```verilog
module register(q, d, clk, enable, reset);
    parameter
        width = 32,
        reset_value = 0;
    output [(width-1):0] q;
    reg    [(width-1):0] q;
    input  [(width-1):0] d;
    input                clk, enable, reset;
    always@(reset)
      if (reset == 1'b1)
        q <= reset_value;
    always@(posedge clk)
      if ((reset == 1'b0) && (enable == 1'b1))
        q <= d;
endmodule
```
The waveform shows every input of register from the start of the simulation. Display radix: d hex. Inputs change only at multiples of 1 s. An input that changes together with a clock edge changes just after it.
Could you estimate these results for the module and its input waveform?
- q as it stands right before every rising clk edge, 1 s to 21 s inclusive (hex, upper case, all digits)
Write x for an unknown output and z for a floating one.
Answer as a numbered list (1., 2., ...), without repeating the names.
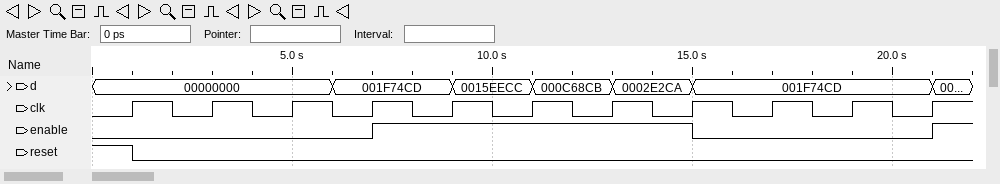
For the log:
1. 00000000, 00000000, 00000000, 00000000, 00000000, 001F74CD, 0015EECC, 000C68CB, 0002E2CA, 0002E2CA, 0002E2CA
